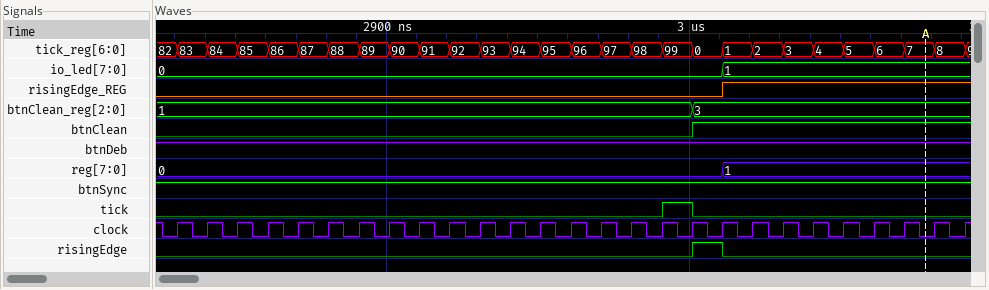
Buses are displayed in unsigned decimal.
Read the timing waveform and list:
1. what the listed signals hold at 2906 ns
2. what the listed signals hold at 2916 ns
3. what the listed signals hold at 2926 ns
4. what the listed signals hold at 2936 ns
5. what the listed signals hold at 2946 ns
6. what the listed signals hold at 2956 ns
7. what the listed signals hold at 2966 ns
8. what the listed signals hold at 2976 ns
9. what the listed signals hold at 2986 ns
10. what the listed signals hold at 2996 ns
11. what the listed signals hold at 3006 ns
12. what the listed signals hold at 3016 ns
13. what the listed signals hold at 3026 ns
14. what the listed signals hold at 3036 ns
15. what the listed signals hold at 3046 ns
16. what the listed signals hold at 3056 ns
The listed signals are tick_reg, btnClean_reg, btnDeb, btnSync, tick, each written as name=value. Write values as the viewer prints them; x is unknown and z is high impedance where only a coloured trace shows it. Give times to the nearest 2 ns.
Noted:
tick_reg=90, btnClean_reg=1, btnDeb=1, btnSync=1, tick=0
tick_reg=91, btnClean_reg=1, btnDeb=1, btnSync=1, tick=0
tick_reg=92, btnClean_reg=1, btnDeb=1, btnSync=1, tick=0
tick_reg=93, btnClean_reg=1, btnDeb=1, btnSync=1, tick=0
tick_reg=94, btnClean_reg=1, btnDeb=1, btnSync=1, tick=0
tick_reg=95, btnClean_reg=1, btnDeb=1, btnSync=1, tick=0
tick_reg=96, btnClean_reg=1, btnDeb=1, btnSync=1, tick=0
tick_reg=97, btnClean_reg=1, btnDeb=1, btnSync=1, tick=0
tick_reg=98, btnClean_reg=1, btnDeb=1, btnSync=1, tick=0
tick_reg=99, btnClean_reg=1, btnDeb=1, btnSync=1, tick=1
tick_reg=0, btnClean_reg=3, btnDeb=1, btnSync=1, tick=0
tick_reg=1, btnClean_reg=3, btnDeb=1, btnSync=1, tick=0
tick_reg=2, btnClean_reg=3, btnDeb=1, btnSync=1, tick=0
tick_reg=3, btnClean_reg=3, btnDeb=1, btnSync=1, tick=0
tick_reg=4, btnClean_reg=3, btnDeb=1, btnSync=1, tick=0
tick_reg=5, btnClean_reg=3, btnDeb=1, btnSync=1, tick=0
